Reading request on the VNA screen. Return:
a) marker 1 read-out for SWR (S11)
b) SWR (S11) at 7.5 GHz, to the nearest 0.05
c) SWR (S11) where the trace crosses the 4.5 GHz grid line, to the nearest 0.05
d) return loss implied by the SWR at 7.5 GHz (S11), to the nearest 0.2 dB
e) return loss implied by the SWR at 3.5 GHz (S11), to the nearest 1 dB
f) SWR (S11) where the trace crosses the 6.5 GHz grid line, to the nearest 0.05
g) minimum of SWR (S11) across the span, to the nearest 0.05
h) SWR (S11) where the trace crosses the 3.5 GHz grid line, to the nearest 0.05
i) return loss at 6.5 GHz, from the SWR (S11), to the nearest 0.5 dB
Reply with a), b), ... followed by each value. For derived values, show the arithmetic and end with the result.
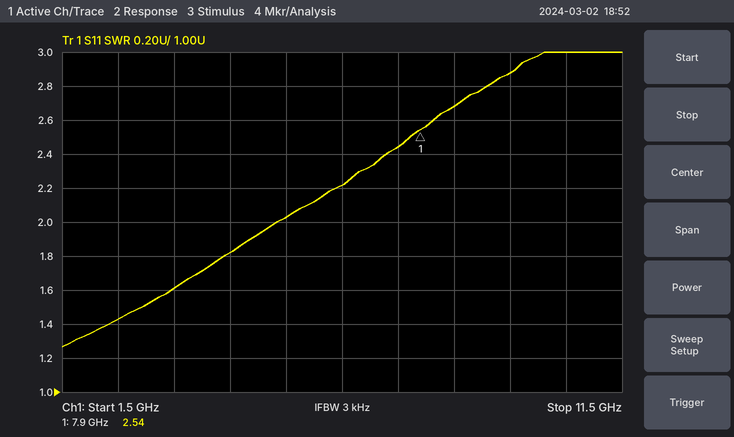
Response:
a) 2.54
b) 2.45
c) 1.80
d) −20 log10((2.45 − 1)/(2.45 + 1)) ≈ 7.53 dB, so 7.6 dB to the nearest 0.2 dB
e) −20 log10((1.6 − 1)/(1.6 + 1)) ≈ 13 dB
f) 2.20
g) 1.25
h) 1.60
i) −20 log10((2.2 − 1)/(2.2 + 1)) ≈ 8.5 dB
